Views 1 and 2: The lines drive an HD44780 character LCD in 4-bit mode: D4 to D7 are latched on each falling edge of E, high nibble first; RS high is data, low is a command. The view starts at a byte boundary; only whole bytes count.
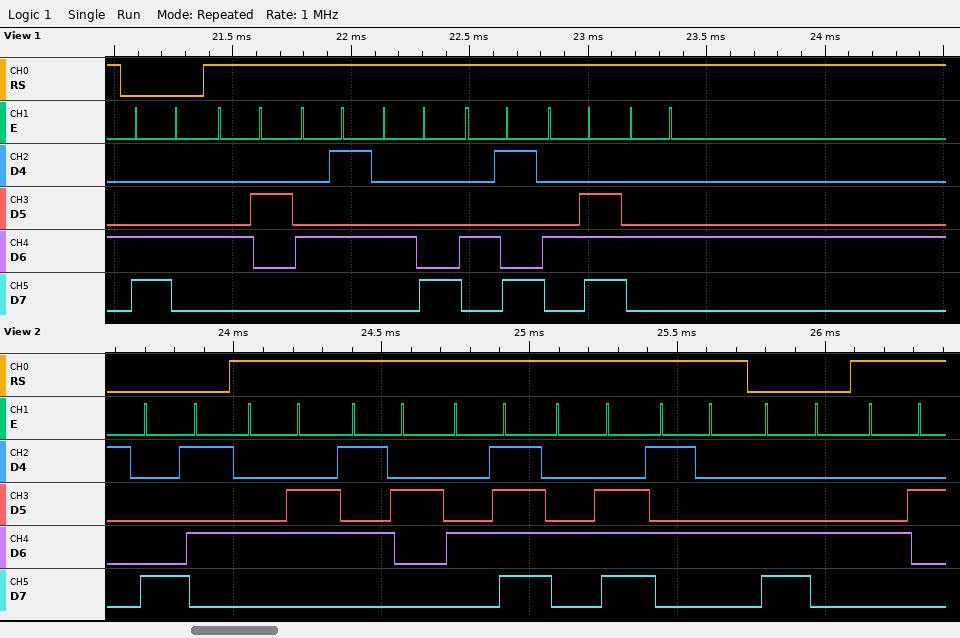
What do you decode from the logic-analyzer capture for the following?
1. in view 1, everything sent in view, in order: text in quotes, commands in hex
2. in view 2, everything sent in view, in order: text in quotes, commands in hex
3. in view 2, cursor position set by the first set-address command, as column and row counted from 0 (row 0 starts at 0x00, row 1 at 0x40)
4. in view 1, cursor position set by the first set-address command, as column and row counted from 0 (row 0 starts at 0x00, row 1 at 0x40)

0xC4 "BEHIND"
0x85 "FRONT" 0xC4 "B"
column 5, row 0
column 4, row 1
